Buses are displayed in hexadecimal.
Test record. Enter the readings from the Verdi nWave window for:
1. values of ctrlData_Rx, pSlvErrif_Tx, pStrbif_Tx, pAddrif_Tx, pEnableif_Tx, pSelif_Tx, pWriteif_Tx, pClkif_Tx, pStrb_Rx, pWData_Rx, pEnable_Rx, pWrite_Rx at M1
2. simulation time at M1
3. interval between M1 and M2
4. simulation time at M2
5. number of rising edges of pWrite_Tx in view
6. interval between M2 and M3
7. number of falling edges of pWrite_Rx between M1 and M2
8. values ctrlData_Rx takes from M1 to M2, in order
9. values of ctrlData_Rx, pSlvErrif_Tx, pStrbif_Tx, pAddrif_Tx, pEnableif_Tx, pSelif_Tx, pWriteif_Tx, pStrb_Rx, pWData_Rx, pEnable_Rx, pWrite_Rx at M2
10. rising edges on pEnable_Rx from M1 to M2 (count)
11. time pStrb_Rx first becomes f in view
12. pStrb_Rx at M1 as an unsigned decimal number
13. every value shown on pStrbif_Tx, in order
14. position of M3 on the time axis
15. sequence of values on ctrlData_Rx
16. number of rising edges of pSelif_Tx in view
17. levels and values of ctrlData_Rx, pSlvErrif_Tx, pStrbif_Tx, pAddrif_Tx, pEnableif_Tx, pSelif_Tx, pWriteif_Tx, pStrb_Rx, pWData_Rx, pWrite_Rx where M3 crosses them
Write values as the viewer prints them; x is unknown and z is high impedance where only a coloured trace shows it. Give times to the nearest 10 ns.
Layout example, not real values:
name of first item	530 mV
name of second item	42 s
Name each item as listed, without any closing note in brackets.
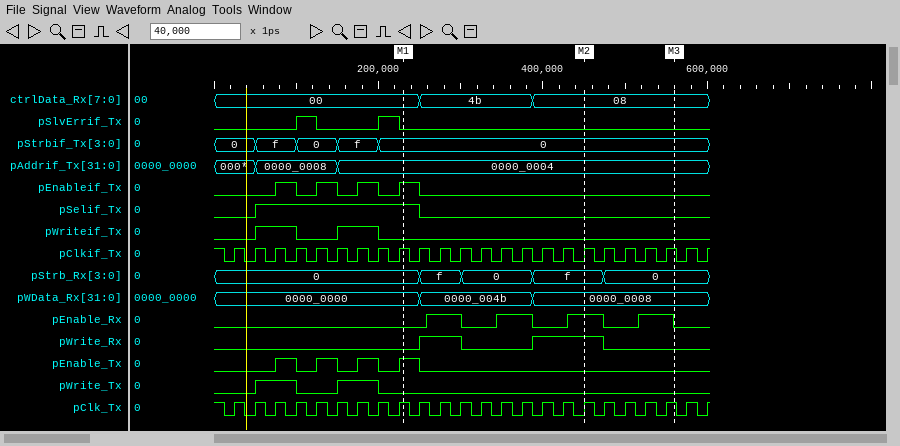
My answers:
values of ctrlData_Rx, pSlvErrif_Tx, pStrbif_Tx, pAddrif_Tx, pEnableif_Tx, pSelif_Tx, pWriteif_Tx, pClkif_Tx, pStrb_Rx, pWData_Rx, pEnable_Rx, pWrite_Rx at M1	ctrlData_Rx=00, pSlvErrif_Tx=0, pStrbif_Tx=0, pAddrif_Tx=0000_0004, pEnableif_Tx=1, pSelif_Tx=1, pWriteif_Tx=0, pClkif_Tx=1, pStrb_Rx=0, pWData_Rx=0000_0000, pEnable_Rx=0, pWrite_Rx=0
simulation time at M1	230 ns
interval between M1 and M2	220 ns
simulation time at M2	450 ns
number of rising edges of pWrite_Tx in view	2
interval between M2 and M3	110 ns
number of falling edges of pWrite_Rx between M1 and M2	1
values ctrlData_Rx takes from M1 to M2, in order	00, 4b, 08
values of ctrlData_Rx, pSlvErrif_Tx, pStrbif_Tx, pAddrif_Tx, pEnableif_Tx, pSelif_Tx, pWriteif_Tx, pStrb_Rx, pWData_Rx, pEnable_Rx, pWrite_Rx at M2	ctrlData_Rx=08, pSlvErrif_Tx=0, pStrbif_Tx=0, pAddrif_Tx=0000_0004, pEnableif_Tx=0, pSelif_Tx=0, pWriteif_Tx=0, pStrb_Rx=f, pWData_Rx=0000_0008, pEnable_Rx=1, pWrite_Rx=1
rising edges on pEnable_Rx from M1 to M2	3
time pStrb_Rx first becomes f in view	250 ns
pStrb_Rx at M1 as an unsigned decimal number	0
every value shown on pStrbif_Tx, in order	0, f, 0, f, 0
position of M3 on the time axis	560 ns
sequence of values on ctrlData_Rx	00, 4b, 08
number of rising edges of pSelif_Tx in view	1
levels and values of ctrlData_Rx, pSlvErrif_Tx, pStrbif_Tx, pAddrif_Tx, pEnableif_Tx, pSelif_Tx, pWriteif_Tx, pStrb_Rx, pWData_Rx, pWrite_Rx where M3 crosses them	ctrlData_Rx=08, pSlvErrif_Tx=0, pStrbif_Tx=0, pAddrif_Tx=0000_0004, pEnableif_Tx=0, pSelif_Tx=0, pWriteif_Tx=0, pStrb_Rx=0, pWData_Rx=0000_0008, pWrite_Rx=0
